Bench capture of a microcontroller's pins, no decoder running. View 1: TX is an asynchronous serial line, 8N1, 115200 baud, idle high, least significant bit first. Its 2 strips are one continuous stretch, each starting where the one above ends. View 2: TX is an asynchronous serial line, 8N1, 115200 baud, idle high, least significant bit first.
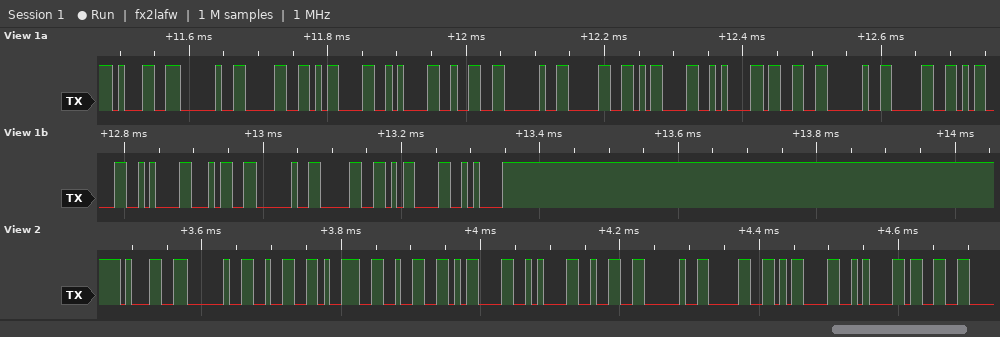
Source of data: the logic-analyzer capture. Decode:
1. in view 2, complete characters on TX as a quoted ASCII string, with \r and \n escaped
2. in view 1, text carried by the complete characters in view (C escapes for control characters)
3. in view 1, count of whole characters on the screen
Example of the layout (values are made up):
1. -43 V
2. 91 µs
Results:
1. "1 292\r\n2 0\r\n3"
2. "1 0\r\n2 0\r\n3 0\r\n4 0\r\n"
3. 20
